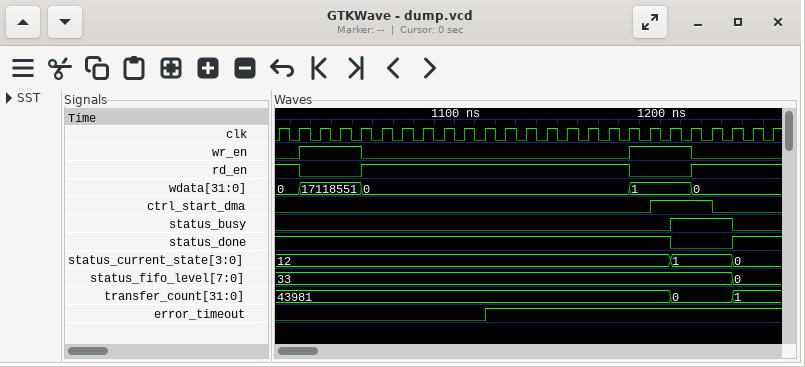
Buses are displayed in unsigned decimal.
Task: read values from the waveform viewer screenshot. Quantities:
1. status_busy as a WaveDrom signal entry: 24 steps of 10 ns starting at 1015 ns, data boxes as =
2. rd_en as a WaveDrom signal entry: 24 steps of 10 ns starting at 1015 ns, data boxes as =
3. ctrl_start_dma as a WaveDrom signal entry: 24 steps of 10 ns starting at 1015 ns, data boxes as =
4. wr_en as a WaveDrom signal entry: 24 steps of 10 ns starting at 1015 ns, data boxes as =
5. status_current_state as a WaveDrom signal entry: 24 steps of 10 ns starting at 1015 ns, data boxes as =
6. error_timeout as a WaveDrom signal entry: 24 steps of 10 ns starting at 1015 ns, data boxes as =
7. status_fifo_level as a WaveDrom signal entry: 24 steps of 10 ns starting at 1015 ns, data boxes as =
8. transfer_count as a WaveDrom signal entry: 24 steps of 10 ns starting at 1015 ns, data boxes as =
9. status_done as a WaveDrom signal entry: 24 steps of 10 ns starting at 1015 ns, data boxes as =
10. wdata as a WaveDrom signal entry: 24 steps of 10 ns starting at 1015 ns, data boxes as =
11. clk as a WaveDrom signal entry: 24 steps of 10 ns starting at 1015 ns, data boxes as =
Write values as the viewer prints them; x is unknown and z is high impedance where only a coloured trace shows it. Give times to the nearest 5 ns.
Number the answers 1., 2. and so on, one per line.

1. {name: 'status_busy', wave: '0..................1..0.'}
2. {name: 'rd_en', wave: '10..1............0..1...'}
3. {name: 'ctrl_start_dma', wave: '0.................1..0..'}
4. {name: 'wr_en', wave: '01..0............1..0...'}
5. {name: 'status_current_state', wave: '=..................=..=.', data: '12 1 0'}
6. {name: 'error_timeout', wave: '0.........1.............'}
7. {name: 'status_fifo_level', wave: '=.....................=.', data: '33 0'}
8. {name: 'transfer_count', wave: '=..................=..=.', data: '43981 0 1'}
9. {name: 'status_done', wave: '1..................0..1.'}
10. {name: 'wdata', wave: '==..=............=..=...', data: '0 17118551 0 1 0'}
11. {name: 'clk', wave: 'p.......................'}
